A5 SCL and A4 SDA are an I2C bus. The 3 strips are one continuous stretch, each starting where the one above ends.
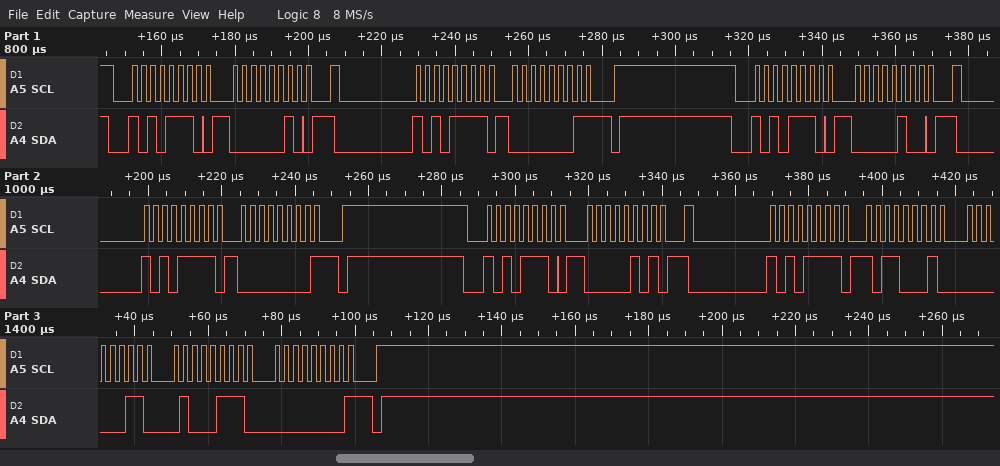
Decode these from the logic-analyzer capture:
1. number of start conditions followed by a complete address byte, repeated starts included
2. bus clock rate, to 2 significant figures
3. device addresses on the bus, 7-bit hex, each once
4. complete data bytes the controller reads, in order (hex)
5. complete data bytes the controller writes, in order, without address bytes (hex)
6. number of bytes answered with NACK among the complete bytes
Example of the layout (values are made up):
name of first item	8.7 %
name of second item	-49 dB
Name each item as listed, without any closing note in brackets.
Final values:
number of start conditions followed by a complete address byte, repeated starts included	6
bus clock rate, to 2 significant figures	400 kHz
device addresses on the bus, 7-bit hex, each once	0x57
complete data bytes the controller reads, in order	01 00 B1 03 47 00
complete data bytes the controller writes, in order, without address bytes	02 04 05
number of bytes answered with NACK among the complete bytes	3
